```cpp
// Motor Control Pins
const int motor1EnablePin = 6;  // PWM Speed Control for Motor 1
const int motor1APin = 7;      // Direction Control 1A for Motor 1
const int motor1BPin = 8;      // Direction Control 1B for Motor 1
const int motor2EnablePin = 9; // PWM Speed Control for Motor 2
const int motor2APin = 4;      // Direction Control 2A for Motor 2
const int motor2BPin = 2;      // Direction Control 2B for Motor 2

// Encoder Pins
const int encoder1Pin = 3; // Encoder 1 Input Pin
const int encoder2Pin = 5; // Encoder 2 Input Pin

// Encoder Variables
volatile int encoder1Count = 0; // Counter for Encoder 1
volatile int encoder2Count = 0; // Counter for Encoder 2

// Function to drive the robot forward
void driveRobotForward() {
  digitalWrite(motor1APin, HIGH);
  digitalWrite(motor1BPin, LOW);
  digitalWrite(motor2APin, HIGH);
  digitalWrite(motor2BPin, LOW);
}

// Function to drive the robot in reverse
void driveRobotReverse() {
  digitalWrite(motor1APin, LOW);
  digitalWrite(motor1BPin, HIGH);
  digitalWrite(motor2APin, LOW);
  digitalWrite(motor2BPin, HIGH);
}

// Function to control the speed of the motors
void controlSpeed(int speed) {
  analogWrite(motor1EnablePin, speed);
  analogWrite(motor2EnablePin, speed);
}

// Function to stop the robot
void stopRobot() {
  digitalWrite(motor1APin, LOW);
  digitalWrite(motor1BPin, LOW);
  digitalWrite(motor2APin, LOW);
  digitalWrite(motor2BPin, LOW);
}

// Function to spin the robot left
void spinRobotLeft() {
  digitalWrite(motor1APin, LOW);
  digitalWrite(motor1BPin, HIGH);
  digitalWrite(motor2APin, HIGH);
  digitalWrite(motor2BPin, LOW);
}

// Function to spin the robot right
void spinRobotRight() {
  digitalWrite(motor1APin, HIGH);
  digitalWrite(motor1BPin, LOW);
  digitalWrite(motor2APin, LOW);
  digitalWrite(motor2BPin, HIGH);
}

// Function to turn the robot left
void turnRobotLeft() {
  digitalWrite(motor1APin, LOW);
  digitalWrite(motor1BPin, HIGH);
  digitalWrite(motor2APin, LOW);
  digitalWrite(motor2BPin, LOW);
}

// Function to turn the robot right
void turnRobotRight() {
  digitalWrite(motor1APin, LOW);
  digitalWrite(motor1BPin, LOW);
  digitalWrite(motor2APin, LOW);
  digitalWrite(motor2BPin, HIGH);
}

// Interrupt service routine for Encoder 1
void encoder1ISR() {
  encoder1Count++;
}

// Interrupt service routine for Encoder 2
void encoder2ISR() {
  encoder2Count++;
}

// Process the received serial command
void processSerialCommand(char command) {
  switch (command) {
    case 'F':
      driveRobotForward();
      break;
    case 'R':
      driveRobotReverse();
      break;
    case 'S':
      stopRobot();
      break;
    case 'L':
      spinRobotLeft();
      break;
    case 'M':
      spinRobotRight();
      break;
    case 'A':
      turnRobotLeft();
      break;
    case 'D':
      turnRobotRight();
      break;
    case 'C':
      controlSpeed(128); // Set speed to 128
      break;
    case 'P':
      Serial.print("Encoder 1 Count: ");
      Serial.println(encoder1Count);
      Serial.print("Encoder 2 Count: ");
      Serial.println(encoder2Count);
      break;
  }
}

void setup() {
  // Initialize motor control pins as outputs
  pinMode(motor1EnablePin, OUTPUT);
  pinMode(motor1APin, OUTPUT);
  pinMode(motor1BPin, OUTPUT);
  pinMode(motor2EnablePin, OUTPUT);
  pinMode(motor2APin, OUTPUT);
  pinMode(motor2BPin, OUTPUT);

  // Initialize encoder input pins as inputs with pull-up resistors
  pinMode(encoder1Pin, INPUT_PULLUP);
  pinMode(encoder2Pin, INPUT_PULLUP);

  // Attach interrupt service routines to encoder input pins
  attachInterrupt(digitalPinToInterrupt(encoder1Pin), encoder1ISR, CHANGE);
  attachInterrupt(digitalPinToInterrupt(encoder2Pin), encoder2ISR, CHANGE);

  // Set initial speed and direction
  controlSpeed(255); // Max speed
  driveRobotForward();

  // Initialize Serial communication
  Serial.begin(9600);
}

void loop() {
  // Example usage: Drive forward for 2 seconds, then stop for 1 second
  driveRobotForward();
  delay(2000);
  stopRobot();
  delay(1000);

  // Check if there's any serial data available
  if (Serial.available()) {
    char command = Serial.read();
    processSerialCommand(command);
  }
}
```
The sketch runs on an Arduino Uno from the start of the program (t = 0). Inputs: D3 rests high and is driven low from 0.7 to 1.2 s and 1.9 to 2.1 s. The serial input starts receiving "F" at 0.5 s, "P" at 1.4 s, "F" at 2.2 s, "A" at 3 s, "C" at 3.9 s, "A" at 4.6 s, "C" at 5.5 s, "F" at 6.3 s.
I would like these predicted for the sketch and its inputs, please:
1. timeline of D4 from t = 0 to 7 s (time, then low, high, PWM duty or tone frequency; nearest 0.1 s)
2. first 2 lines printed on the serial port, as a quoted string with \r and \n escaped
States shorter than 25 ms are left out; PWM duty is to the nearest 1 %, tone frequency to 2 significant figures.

0 s high; 2 s low; 3 s high; 5 s low; 6 s high
"Encoder 1 Count: 4\r\nEncoder 2 Count: 0\r\n"
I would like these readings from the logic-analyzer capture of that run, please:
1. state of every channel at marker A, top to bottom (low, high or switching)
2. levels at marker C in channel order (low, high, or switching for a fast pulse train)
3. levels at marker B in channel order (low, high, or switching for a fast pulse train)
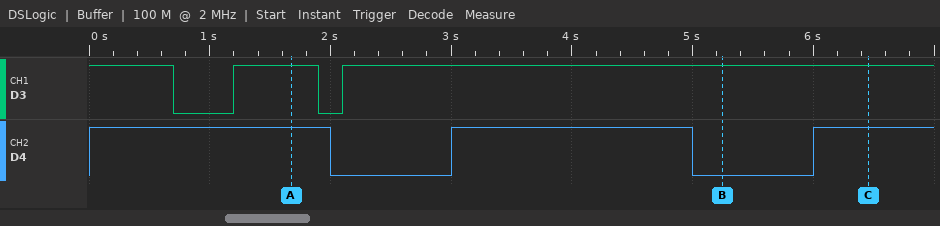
D3 high, D4 high
D3 high, D4 high
D3 high, D4 low
